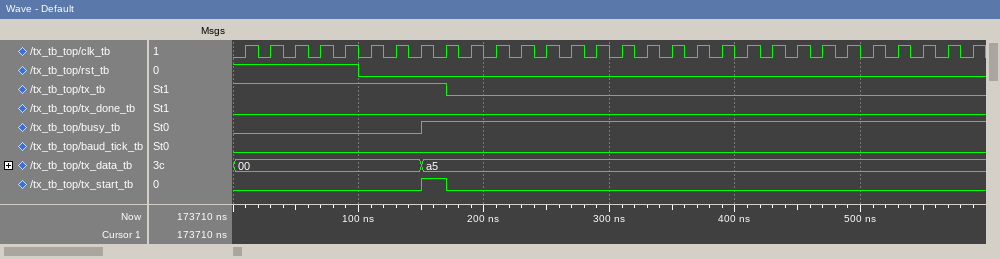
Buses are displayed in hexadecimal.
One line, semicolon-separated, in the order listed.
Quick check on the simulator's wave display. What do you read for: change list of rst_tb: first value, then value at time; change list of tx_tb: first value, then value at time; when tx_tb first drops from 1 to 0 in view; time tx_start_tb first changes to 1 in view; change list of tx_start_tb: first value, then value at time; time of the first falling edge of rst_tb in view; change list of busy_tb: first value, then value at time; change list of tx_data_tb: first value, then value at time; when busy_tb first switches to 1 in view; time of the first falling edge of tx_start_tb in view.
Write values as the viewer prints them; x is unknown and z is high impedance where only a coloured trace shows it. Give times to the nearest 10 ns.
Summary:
1, 0 at 100 ns; 1, 0 at 170 ns; 170 ns; 150 ns; 0, 1 at 150 ns, 0 at 170 ns; 100 ns; 0, 1 at 150 ns; 00, a5 at 150 ns; 150 ns; 170 ns
